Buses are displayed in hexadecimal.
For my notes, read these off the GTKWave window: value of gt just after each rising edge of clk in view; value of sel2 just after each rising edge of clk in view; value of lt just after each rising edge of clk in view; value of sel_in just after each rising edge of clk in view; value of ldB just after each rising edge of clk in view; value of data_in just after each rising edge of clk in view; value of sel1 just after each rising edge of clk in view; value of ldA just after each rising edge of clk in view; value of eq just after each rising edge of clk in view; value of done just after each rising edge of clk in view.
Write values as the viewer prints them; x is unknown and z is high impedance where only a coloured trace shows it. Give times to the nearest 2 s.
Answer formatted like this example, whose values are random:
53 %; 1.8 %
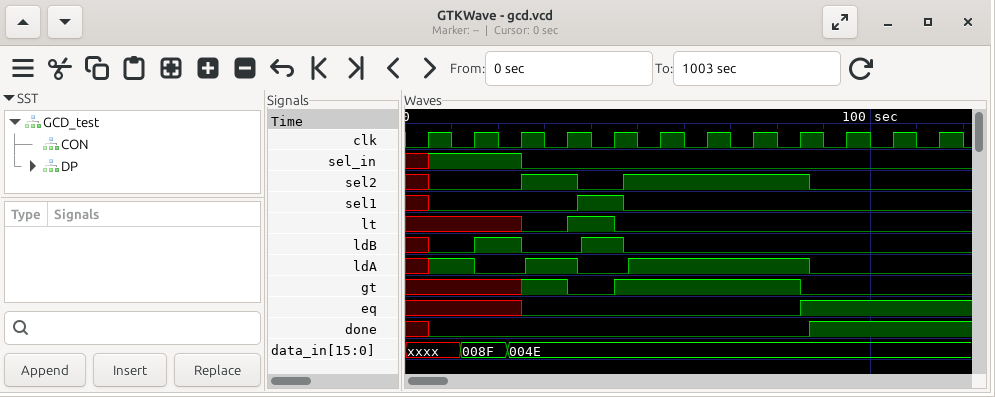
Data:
x x 1 0 1 1 1 1 0 0 0 0; 0 0 1 1 0 1 1 1 1 0 0 0; x x 0 1 0 0 0 0 0 0 0 0; 1 1 0 0 0 0 0 0 0 0 0 0; 0 1 0 0 1 0 0 0 0 0 0 0; xxxx, 008F, 004E, 004E, 004E, 004E, 004E, 004E, 004E, 004E, 004E, 004E; 0 0 0 0 1 0 0 0 0 0 0 0; 1 0 0 1 0 1 1 1 1 0 0 0; x x 0 0 0 0 0 0 1 1 1 1; 0 0 0 0 0 0 0 0 0 1 1 1
